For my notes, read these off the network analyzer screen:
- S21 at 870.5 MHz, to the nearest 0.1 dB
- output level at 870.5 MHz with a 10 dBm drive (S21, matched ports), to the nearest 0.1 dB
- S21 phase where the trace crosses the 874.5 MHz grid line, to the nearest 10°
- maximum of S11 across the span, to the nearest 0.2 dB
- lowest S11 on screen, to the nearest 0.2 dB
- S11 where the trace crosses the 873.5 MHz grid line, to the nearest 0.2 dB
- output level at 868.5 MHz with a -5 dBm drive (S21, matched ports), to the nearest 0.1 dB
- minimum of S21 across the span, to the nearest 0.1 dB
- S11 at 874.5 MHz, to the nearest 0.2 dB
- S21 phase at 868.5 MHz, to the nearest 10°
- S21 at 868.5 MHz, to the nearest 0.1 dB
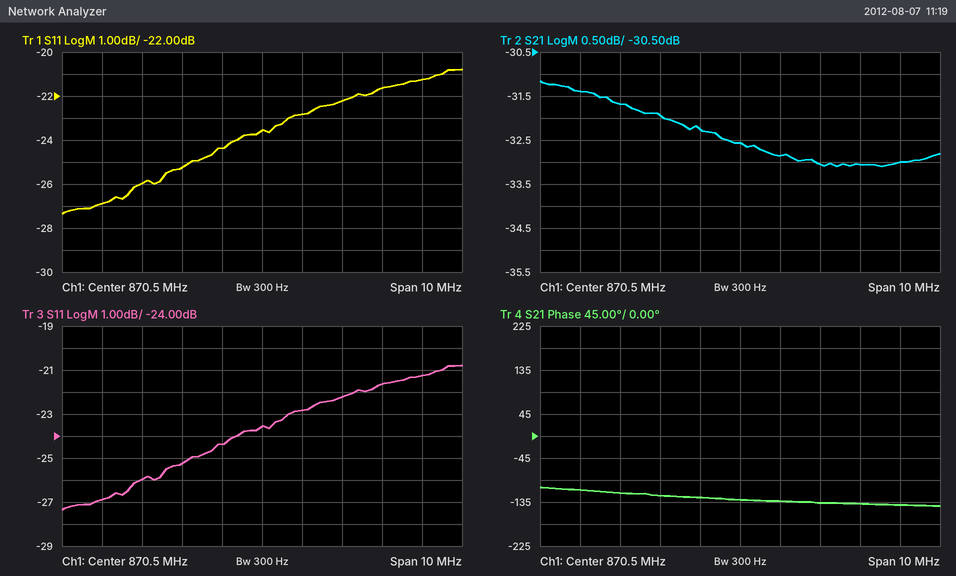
-32.6 dB
-22.6 dBm
-140°
-20.8 dB
-27.4 dB
-21.6 dB
-36.9 dBm
-33.1 dB
-21.2 dB
-120°
-31.9 dB
